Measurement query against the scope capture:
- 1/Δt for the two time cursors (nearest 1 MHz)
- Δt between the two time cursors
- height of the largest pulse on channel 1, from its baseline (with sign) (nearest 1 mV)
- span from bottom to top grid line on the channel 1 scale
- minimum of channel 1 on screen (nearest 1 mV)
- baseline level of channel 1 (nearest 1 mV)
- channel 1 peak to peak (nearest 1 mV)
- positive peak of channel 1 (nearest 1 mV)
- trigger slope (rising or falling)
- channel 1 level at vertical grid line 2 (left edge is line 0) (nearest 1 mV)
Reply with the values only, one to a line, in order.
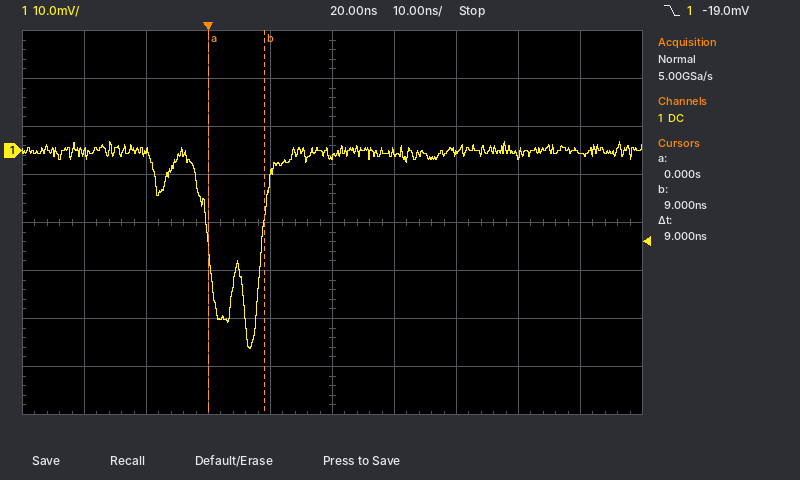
111 MHz
9 ns
-41 mV
80 mV
-41 mV
0 mV
43 mV
2 mV
falling
0 mV
